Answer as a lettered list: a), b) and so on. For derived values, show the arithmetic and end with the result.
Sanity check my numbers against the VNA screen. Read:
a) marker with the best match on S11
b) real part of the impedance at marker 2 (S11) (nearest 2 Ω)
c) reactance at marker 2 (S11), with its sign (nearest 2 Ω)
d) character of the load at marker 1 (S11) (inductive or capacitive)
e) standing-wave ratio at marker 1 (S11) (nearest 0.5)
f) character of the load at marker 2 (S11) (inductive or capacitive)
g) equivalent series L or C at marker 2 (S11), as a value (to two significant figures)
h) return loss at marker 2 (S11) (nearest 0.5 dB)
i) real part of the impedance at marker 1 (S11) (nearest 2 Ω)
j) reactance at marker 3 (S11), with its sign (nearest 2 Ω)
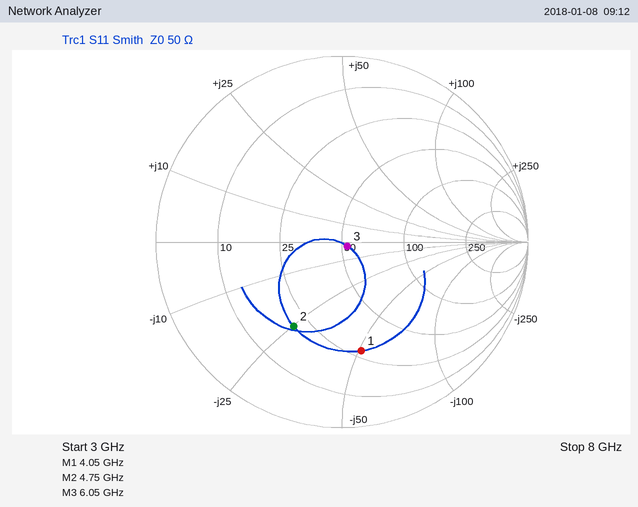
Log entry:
a) marker 3
b) 20 Ω
c) -26 Ω
d) capacitive
e) 4.0
f) capacitive
g) C = 1/(2π × 4.75 GHz × 26 Ω) ≈ 1.3 pF
h) 5.5 dB
i) 28 Ω
j) -2 Ω
